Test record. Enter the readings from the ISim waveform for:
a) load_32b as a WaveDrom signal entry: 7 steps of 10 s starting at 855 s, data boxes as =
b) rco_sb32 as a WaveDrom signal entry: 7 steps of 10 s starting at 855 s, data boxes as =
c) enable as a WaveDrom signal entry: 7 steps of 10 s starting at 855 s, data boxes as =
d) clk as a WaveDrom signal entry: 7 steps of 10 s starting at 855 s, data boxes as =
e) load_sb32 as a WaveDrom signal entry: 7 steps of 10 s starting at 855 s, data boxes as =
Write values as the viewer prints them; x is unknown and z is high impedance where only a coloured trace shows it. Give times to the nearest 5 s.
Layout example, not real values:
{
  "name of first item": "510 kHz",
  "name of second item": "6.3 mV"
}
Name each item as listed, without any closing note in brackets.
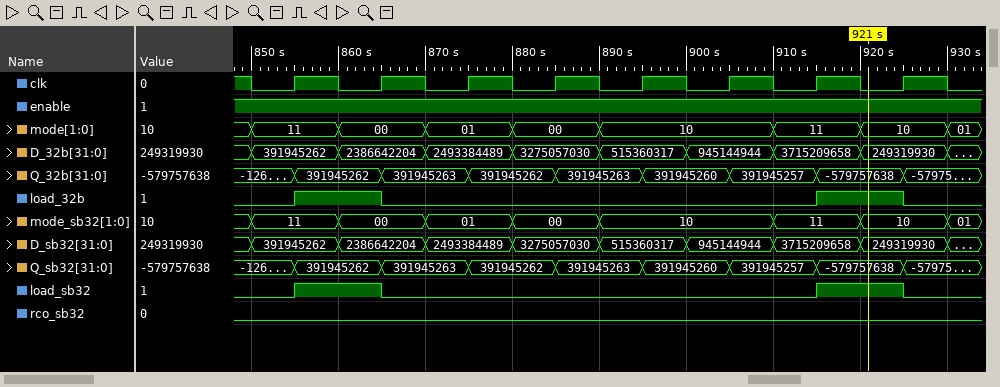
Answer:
{
  "load_32b as a WaveDrom signal entry: 7 steps of 10 s starting at 855 s, data boxes as =": "{name: 'load_32b', wave: '10....1'}",
  "rco_sb32 as a WaveDrom signal entry: 7 steps of 10 s starting at 855 s, data boxes as =": "{name: 'rco_sb32', wave: '0......'}",
  "enable as a WaveDrom signal entry: 7 steps of 10 s starting at 855 s, data boxes as =": "{name: 'enable', wave: '1......'}",
  "clk as a WaveDrom signal entry: 7 steps of 10 s starting at 855 s, data boxes as =": "{name: 'clk', wave: 'p......'}",
  "load_sb32 as a WaveDrom signal entry: 7 steps of 10 s starting at 855 s, data boxes as =": "{name: 'load_sb32', wave: '10....1'}"
}
